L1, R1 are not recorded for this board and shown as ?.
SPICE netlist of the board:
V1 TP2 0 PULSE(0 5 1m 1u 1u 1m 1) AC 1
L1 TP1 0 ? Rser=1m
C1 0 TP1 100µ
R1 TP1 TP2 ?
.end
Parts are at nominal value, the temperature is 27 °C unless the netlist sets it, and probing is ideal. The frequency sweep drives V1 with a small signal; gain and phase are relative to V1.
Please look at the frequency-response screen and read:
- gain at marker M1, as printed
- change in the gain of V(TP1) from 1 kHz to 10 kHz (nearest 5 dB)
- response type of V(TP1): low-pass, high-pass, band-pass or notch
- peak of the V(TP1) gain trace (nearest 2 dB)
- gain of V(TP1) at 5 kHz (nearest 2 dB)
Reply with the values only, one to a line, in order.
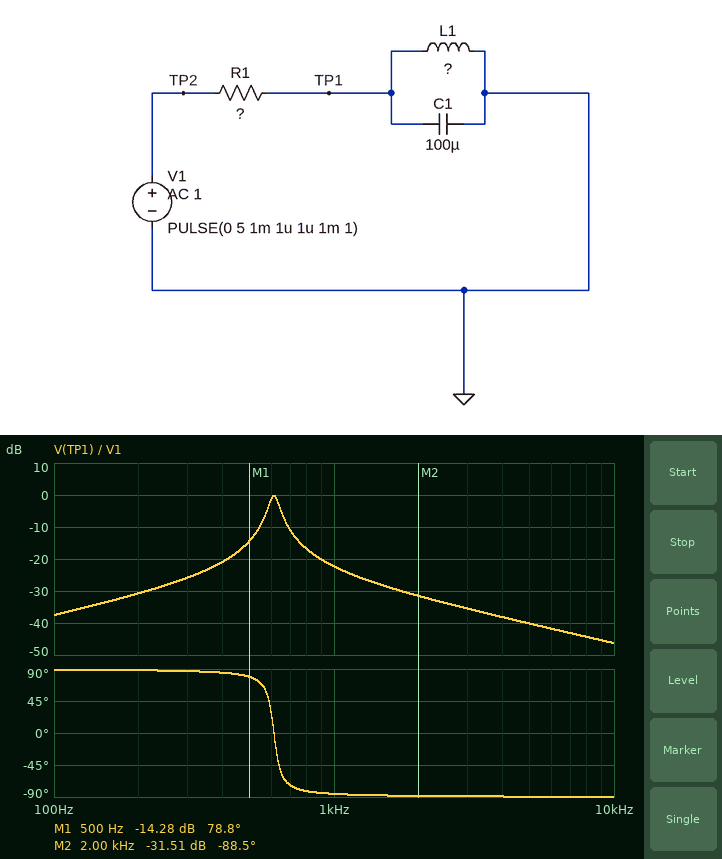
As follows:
-14.28 dB
-25 dB
band-pass
0 dB
-40 dB
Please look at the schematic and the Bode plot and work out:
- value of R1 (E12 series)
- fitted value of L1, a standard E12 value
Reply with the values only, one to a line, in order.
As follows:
33 Ω
680 µH
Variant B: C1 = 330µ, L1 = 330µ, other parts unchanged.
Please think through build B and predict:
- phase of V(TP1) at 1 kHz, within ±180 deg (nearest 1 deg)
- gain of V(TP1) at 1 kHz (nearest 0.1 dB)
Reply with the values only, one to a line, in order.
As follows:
-89 deg
-34.4 dB
